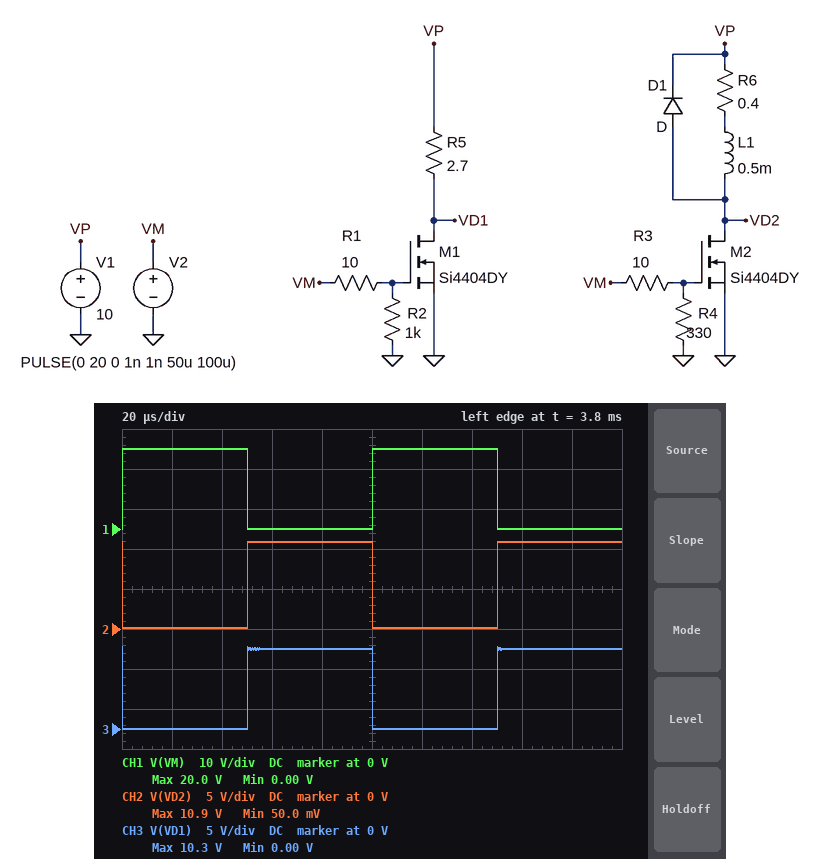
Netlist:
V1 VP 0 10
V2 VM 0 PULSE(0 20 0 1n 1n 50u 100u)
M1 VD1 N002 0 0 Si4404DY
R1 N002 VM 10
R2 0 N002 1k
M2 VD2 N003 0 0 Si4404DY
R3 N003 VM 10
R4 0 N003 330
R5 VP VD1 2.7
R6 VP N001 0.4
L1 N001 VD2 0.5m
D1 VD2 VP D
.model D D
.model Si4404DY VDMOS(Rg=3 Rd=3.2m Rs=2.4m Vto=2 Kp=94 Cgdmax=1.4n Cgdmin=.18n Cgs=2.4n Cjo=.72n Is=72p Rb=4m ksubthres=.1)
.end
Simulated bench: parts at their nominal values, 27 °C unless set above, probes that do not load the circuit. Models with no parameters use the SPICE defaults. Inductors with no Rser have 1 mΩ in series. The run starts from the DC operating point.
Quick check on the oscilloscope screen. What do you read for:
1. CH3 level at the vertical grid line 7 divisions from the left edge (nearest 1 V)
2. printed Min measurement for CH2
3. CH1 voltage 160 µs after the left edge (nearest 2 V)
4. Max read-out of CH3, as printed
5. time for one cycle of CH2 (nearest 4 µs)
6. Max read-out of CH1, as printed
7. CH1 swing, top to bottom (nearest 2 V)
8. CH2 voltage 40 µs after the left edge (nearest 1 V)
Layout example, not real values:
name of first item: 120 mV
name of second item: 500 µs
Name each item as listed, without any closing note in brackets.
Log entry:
CH3 level at the vertical grid line 7 divisions from the left edge: 0 V
printed Min measurement for CH2: 50.0 mV
CH1 voltage 160 µs after the left edge: 0 V
Max read-out of CH3, as printed: 10.3 V
time for one cycle of CH2: 100 µs
Max read-out of CH1, as printed: 20.0 V
CH1 swing, top to bottom: 20 V
CH2 voltage 40 µs after the left edge: 0 V
